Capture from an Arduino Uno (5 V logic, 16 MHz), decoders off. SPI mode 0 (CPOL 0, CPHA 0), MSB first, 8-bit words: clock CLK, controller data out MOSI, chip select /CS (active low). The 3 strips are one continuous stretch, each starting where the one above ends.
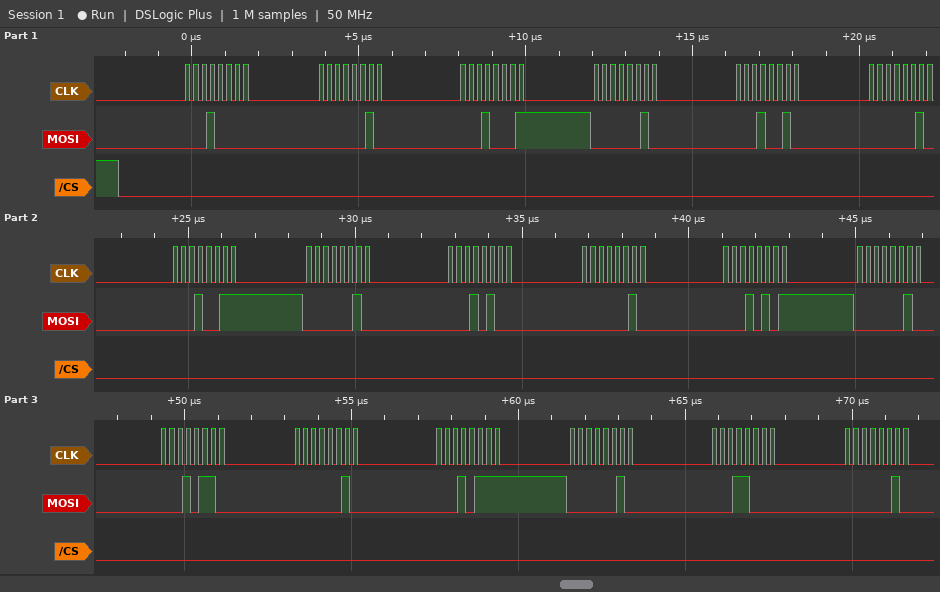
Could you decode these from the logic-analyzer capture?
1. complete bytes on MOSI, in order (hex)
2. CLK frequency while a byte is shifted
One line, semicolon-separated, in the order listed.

10 02 11 02 12 02 13 02 14 02 15 02 16 02 17 02 18 02; 4 MHz
